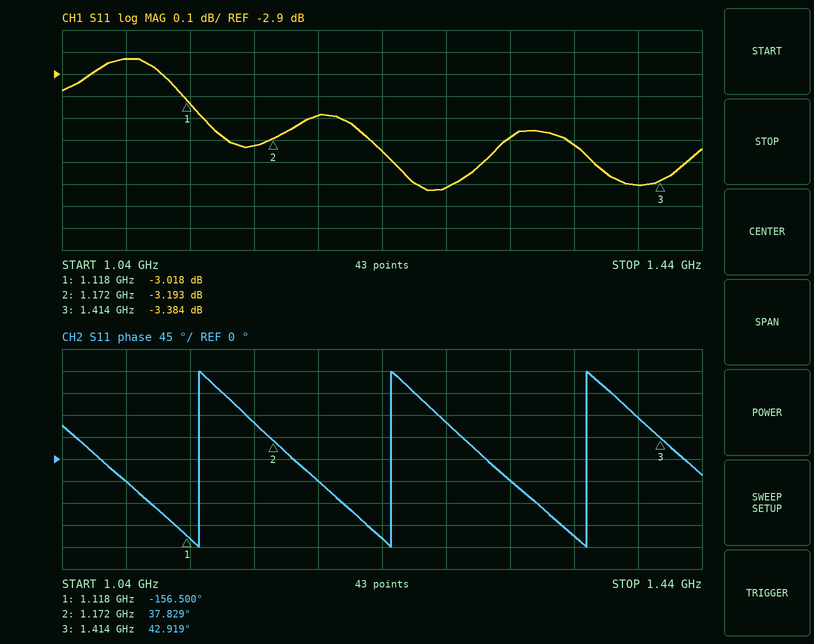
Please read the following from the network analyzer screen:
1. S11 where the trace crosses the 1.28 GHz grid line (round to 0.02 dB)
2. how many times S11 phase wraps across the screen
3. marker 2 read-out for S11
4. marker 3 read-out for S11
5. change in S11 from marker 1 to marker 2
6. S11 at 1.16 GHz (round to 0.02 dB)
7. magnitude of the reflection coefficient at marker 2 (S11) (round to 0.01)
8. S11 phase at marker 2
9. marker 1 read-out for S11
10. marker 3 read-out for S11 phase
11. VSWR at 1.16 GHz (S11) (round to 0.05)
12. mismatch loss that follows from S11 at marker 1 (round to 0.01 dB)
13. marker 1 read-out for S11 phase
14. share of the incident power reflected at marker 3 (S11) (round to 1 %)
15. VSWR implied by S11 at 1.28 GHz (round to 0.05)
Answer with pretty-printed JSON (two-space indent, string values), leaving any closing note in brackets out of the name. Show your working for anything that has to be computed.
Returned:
{
  "S11 where the trace crosses the 1.28 GHz grid line": "-3.42 dB",
  "how many times S11 phase wraps across the screen": "3",
  "marker 2 read-out for S11": "-3.193 dB",
  "marker 3 read-out for S11": "-3.384 dB",
  "change in S11 from marker 1 to marker 2": "-3.193 − (-3.018) = -0.175 dB",
  "S11 at 1.16 GHz": "-3.22 dB",
  "magnitude of the reflection coefficient at marker 2 (S11)": "10^(-3.193/20) ≈ 0.69",
  "S11 phase at marker 2": "37.829°",
  "marker 1 read-out for S11": "-3.018 dB",
  "marker 3 read-out for S11 phase": "42.919°",
  "VSWR at 1.16 GHz (S11)": "|Γ| = 10^(-3.22/20) = 0.6902; VSWR = (1 + 0.6902)/(1 − 0.6902) ≈ 5.46, so 5.45 to the nearest 0.05",
  "mismatch loss that follows from S11 at marker 1": "−10 log10(1 − 10^(-3.018/10)) ≈ 3.00 dB",
  "marker 1 read-out for S11 phase": "-156.500°",
  "share of the incident power reflected at marker 3 (S11)": "10^(-3.384/10) ≈ 46 %",
  "VSWR implied by S11 at 1.28 GHz": "|Γ| = 10^(-3.42/20) = 0.6745; VSWR = (1 + 0.6745)/(1 − 0.6745) ≈ 5.14, so 5.15 to the nearest 0.05"
}
